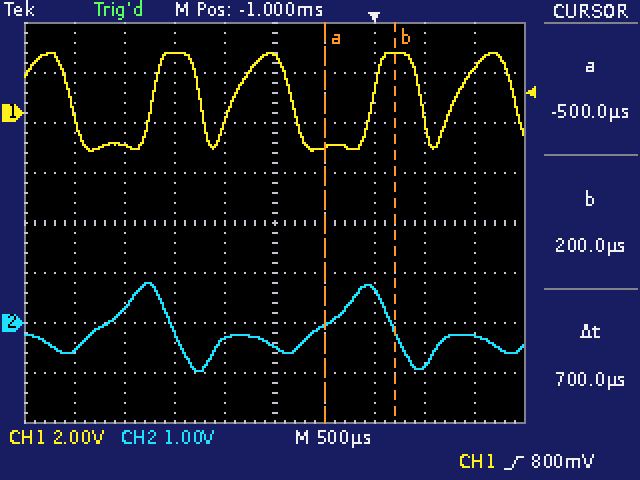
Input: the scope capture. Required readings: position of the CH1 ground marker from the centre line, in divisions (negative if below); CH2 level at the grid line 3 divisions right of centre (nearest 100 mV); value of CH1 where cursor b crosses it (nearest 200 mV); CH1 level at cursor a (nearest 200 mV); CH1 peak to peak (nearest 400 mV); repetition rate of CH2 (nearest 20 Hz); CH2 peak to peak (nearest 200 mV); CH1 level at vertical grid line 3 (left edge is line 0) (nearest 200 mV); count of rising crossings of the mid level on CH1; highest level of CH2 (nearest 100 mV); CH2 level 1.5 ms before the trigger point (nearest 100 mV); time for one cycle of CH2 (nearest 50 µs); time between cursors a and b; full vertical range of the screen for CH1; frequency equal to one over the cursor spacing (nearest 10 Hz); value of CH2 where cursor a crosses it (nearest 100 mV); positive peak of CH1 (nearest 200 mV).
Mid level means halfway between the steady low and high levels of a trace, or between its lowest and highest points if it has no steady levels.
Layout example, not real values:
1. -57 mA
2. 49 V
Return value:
1. +2.2 div
2. -900 mV
3. 2.4 V
4. -1.4 V
5. 4.0 V
6. 460 Hz
7. 1.8 V
8. 2.4 V
9. 4
10. 800 mV
11. -300 mV
12. 2.20 ms
13. 700 µs
14. 16 V
15. 1.43 kHz
16. 0.0 V
17. 2.4 V
